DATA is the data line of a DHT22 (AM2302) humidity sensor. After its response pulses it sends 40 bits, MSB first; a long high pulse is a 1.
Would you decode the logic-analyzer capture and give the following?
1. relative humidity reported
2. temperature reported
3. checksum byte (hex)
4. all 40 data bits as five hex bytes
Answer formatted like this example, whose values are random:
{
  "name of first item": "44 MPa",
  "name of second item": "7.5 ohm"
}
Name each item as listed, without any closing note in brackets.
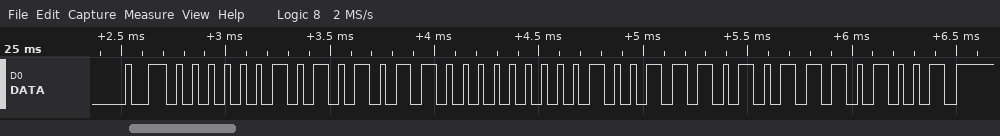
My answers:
{
  "relative humidity reported": "68.4 %",
  "temperature reported": "31.4 °C",
  "checksum byte": "0xE9",
  "all 40 data bits as five hex bytes": "02 AC 01 3A E9"
}
